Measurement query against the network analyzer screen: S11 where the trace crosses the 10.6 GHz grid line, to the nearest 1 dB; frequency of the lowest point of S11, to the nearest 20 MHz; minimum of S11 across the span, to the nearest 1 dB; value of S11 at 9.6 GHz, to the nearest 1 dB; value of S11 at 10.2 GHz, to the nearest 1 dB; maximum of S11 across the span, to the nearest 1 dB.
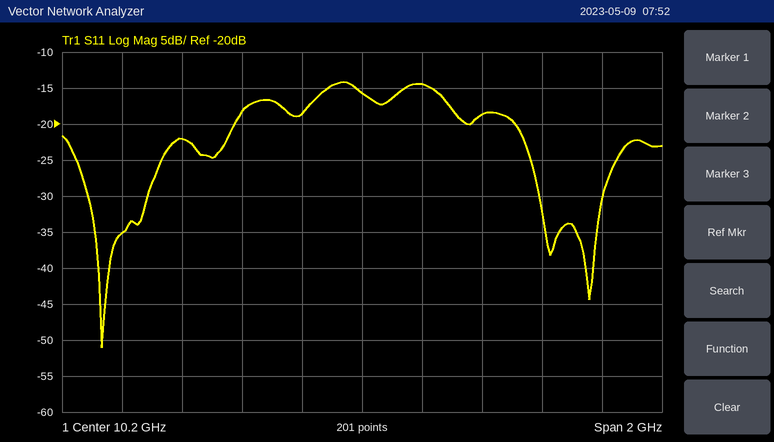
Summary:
-19 dB
9.34 GHz
-51 dB
-22 dB
-16 dB
-14 dB
